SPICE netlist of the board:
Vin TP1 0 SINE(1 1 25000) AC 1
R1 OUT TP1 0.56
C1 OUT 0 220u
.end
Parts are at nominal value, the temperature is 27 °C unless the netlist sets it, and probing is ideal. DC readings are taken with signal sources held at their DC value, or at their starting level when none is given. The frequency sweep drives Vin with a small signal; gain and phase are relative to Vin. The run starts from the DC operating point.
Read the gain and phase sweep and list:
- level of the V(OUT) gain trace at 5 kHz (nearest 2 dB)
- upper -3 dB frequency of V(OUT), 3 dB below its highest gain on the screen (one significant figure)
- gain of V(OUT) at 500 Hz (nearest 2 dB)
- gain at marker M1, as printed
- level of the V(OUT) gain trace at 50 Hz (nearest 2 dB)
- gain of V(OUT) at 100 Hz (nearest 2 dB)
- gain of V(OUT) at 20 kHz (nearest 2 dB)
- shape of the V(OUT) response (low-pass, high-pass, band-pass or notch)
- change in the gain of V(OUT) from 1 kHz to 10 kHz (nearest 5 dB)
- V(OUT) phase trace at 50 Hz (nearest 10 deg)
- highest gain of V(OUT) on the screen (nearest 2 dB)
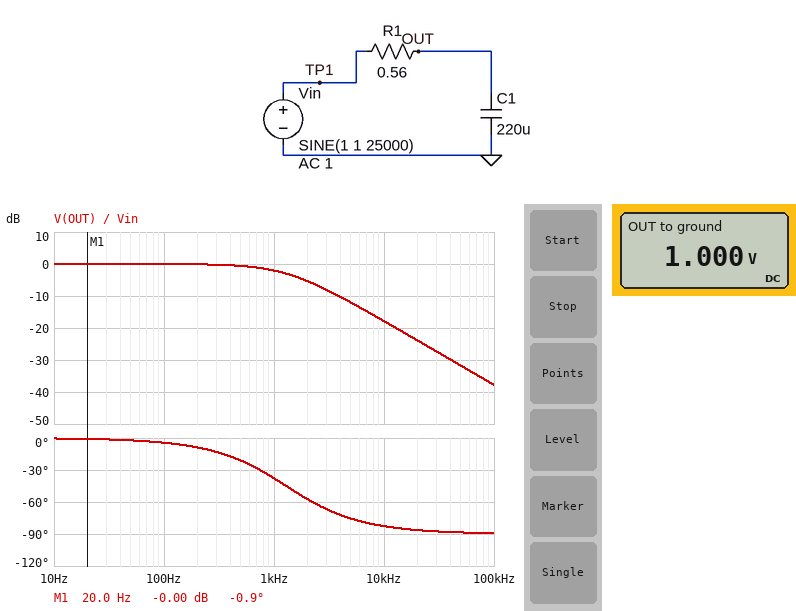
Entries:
-12 dB
1 kHz
0 dB
-0.00 dB
0 dB
0 dB
-24 dB
low-pass
-15 dB
0 deg
0 dB
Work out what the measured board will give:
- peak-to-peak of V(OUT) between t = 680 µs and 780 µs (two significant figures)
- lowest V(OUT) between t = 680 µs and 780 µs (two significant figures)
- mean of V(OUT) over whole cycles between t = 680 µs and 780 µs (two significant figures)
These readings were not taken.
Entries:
100 mV
950 mV
1.0 V
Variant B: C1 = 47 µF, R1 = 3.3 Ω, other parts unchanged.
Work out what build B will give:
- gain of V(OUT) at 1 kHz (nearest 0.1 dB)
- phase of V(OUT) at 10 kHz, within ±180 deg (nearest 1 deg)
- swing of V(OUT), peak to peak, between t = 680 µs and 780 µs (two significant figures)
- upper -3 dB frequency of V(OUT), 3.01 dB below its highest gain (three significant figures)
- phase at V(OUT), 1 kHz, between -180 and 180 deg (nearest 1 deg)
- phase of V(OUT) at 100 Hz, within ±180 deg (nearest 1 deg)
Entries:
-2.9 dB
-84 deg
82 mV
1.03 kHz
-44 deg
-6 deg
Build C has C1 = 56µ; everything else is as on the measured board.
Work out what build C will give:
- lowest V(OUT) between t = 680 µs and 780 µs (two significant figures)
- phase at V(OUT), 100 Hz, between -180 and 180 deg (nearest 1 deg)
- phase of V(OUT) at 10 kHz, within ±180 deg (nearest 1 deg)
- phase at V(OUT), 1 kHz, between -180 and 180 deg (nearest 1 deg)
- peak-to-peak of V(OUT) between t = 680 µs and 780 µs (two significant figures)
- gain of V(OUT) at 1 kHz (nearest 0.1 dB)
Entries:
800 mV
-1 deg
-63 deg
-11 deg
400 mV
-0.2 dB
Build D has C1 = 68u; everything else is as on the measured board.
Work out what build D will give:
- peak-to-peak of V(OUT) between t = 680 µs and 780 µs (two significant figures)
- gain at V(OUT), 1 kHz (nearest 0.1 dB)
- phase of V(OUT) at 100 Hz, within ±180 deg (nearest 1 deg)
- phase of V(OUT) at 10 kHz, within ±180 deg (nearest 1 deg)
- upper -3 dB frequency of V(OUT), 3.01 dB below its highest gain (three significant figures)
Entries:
330 mV
-0.2 dB
-1 deg
-67 deg
4.18 kHz
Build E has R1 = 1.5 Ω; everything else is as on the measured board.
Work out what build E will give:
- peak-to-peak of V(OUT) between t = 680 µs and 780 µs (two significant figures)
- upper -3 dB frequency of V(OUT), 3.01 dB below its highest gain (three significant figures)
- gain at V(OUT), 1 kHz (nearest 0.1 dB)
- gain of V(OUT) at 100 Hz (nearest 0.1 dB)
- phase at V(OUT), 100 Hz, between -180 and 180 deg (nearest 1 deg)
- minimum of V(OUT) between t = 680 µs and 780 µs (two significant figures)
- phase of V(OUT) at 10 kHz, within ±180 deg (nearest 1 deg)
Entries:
39 mV
482 Hz
-7.2 dB
-0.2 dB
-12 deg
980 mV
-87 deg
